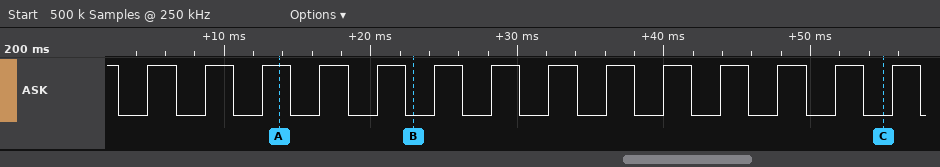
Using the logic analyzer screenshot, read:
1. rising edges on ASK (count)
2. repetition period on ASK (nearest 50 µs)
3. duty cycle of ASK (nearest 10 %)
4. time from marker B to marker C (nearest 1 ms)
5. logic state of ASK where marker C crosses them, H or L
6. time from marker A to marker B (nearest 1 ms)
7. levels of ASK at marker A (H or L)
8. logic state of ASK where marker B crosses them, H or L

14
3900 µs
50 %
32 ms
ASK=L
9 ms
ASK=H
ASK=L
